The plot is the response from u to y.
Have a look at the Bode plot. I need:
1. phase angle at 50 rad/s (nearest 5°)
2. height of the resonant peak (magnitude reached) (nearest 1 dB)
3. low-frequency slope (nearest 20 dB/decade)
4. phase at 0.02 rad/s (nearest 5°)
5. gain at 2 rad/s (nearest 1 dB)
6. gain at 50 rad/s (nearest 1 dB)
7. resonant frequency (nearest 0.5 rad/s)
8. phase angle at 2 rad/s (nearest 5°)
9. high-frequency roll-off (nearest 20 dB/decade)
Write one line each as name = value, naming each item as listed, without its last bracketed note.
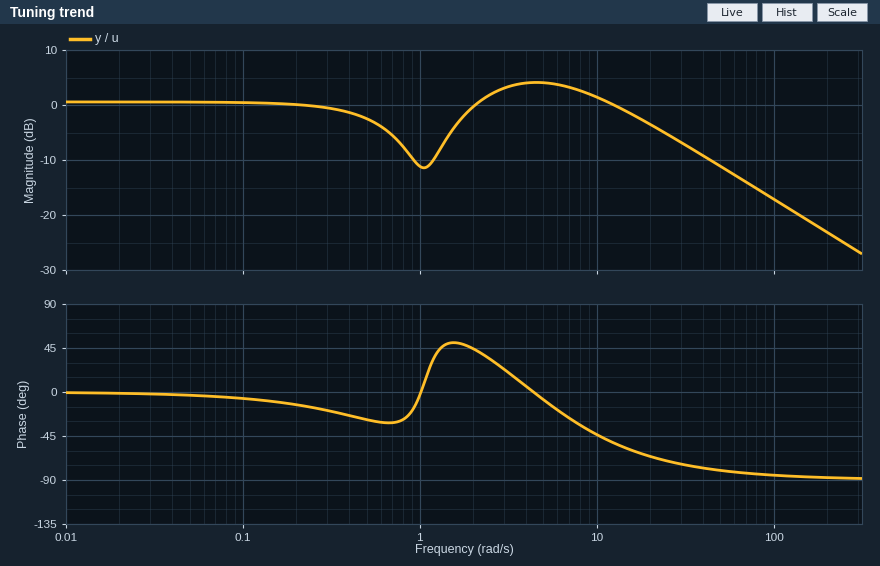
phase angle at 50 rad/s = -80°
height of the resonant peak (magnitude reached) = 4 dB
low-frequency slope = 0 dB/decade
phase at 0.02 rad/s = 0°
gain at 2 rad/s = 0 dB
gain at 50 rad/s = -11 dB
resonant frequency = 4.5 rad/s
phase angle at 2 rad/s = 45°
high-frequency roll-off = -20 dB/decade
